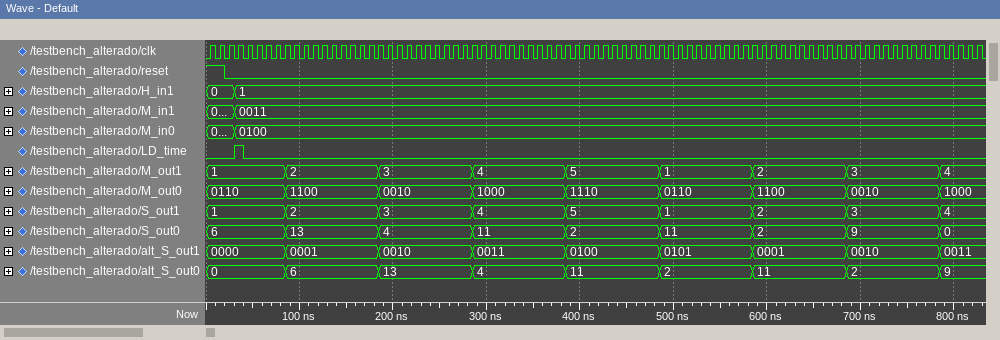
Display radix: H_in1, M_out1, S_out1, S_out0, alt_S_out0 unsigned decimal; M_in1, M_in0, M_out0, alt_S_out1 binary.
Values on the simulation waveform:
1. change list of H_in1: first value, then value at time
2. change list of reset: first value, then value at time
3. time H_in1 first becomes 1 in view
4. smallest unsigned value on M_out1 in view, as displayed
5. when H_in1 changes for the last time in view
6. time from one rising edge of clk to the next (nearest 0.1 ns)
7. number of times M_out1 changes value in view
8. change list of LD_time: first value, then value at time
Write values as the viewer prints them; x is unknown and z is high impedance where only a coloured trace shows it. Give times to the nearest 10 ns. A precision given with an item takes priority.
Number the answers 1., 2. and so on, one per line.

1. 0, 1 at 30 ns
2. 1, 0 at 20 ns
3. 30 ns
4. 1
5. 30 ns
6. 10 ns
7. 8
8. 0, 1 at 30 ns, 0 at 40 ns
